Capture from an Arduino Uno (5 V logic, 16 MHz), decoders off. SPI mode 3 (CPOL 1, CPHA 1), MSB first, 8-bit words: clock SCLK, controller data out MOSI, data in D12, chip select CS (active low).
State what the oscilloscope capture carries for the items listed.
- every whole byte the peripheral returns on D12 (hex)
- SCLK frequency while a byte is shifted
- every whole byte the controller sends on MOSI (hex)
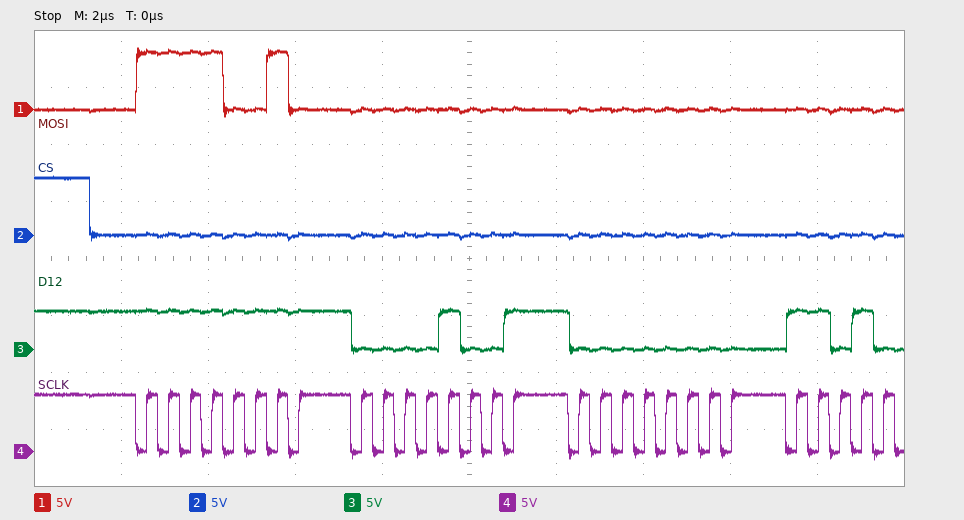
FF 09 00
2 MHz
F2 00 00
